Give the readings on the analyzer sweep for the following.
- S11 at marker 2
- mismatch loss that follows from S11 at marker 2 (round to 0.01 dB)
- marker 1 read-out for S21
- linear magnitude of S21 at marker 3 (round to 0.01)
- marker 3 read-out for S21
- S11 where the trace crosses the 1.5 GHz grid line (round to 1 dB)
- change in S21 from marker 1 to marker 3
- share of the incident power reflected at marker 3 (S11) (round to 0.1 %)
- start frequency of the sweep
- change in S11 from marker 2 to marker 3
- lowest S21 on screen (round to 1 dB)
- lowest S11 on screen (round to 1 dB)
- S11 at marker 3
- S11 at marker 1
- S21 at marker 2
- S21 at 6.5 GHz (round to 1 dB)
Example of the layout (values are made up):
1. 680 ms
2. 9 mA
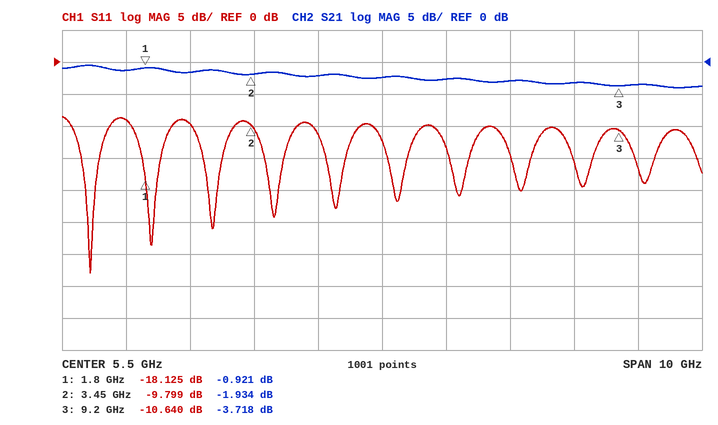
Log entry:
1. -9.799 dB
2. 0.48 dB
3. -0.921 dB
4. 0.65
5. -3.718 dB
6. -9 dB
7. -2.797 dB
8. 8.6 %
9. 500 MHz
10. -0.841 dB
11. -4 dB
12. -33 dB
13. -10.640 dB
14. -18.125 dB
15. -1.934 dB
16. -3 dB
